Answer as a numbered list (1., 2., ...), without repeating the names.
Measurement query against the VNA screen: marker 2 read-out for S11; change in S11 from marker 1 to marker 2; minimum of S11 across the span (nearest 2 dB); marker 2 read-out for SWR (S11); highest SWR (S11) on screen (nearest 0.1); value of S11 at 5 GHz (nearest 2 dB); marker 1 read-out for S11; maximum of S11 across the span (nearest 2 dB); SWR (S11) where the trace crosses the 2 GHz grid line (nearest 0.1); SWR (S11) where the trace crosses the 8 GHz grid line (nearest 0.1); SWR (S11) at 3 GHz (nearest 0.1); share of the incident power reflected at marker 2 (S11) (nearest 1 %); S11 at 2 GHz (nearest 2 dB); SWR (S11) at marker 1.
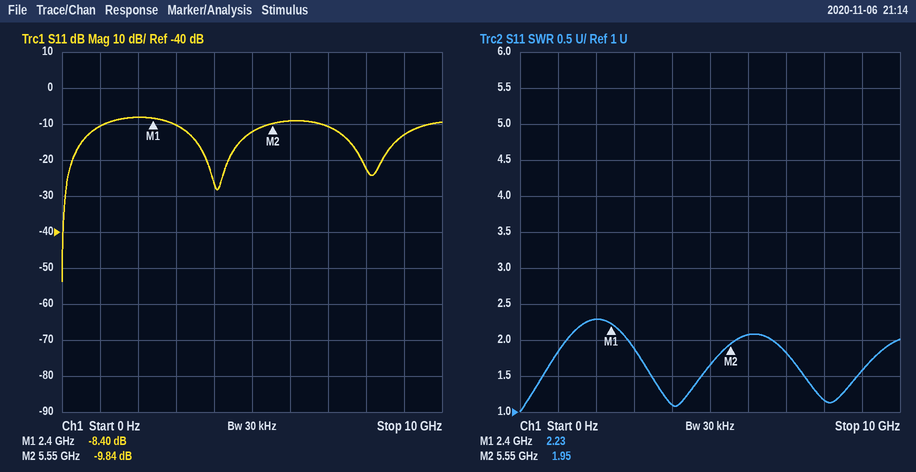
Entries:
1. -9.84 dB
2. -1.44 dB
3. -54 dB
4. 1.95
5. 2.3
6. -12 dB
7. -8.40 dB
8. -8 dB
9. 2.3
10. 1.2
11. 1.9
12. 10 %
13. -8 dB
14. 2.23
